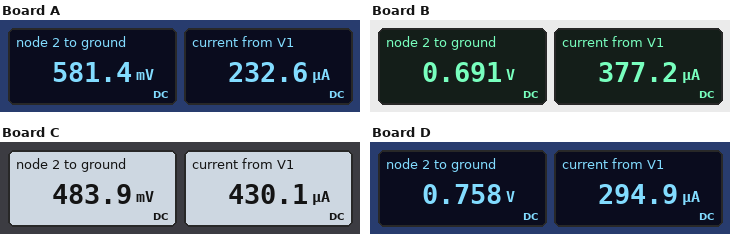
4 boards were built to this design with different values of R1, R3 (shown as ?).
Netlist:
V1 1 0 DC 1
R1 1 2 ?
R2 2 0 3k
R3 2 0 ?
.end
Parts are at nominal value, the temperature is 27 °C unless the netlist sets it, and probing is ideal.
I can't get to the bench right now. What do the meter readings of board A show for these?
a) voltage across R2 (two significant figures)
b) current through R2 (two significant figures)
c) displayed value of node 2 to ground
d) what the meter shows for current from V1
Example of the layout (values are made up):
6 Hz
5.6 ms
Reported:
580 mV
190 µA
581.4 mV
232.6 µA
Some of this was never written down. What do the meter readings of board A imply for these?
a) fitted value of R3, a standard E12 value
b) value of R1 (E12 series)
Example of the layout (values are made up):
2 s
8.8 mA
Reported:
15 kΩ
1.8 kΩ
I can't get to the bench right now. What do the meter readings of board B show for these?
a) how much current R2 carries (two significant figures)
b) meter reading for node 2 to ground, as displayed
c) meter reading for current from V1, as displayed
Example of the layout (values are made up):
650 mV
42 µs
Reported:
230 µA
0.691 V
377.2 µA
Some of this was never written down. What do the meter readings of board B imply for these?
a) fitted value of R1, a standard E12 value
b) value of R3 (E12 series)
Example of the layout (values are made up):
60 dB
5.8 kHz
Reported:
820 Ω
4.7 kΩ
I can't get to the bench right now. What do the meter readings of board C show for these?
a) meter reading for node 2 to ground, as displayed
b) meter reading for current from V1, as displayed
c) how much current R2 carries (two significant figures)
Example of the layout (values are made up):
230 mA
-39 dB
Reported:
483.9 mV
430.1 µA
160 µA
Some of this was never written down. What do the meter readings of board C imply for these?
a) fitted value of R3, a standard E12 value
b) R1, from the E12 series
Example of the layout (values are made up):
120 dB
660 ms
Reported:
1.8 kΩ
1.2 kΩ
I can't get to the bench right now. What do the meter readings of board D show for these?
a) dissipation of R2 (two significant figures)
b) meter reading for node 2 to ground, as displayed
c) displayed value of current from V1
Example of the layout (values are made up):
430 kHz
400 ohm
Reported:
190 µW
0.758 V
294.9 µA
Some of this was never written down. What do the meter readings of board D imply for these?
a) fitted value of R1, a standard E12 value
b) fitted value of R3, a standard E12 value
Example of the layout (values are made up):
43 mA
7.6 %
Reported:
820 Ω
18 kΩ
